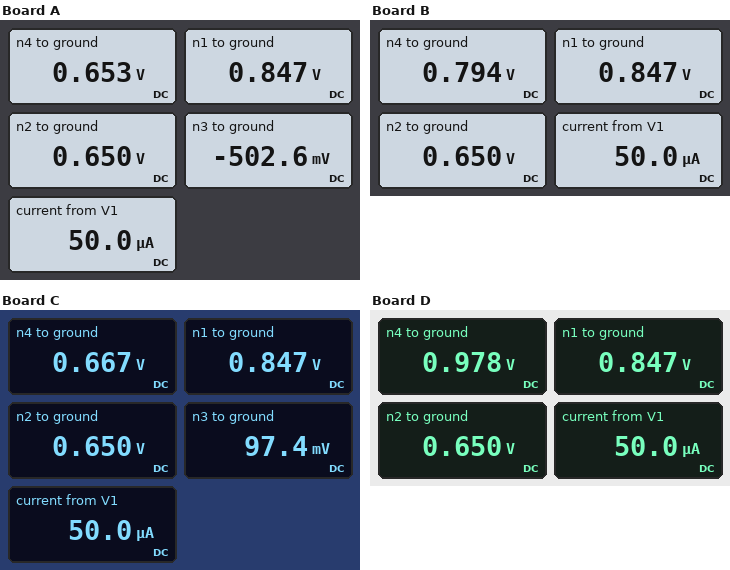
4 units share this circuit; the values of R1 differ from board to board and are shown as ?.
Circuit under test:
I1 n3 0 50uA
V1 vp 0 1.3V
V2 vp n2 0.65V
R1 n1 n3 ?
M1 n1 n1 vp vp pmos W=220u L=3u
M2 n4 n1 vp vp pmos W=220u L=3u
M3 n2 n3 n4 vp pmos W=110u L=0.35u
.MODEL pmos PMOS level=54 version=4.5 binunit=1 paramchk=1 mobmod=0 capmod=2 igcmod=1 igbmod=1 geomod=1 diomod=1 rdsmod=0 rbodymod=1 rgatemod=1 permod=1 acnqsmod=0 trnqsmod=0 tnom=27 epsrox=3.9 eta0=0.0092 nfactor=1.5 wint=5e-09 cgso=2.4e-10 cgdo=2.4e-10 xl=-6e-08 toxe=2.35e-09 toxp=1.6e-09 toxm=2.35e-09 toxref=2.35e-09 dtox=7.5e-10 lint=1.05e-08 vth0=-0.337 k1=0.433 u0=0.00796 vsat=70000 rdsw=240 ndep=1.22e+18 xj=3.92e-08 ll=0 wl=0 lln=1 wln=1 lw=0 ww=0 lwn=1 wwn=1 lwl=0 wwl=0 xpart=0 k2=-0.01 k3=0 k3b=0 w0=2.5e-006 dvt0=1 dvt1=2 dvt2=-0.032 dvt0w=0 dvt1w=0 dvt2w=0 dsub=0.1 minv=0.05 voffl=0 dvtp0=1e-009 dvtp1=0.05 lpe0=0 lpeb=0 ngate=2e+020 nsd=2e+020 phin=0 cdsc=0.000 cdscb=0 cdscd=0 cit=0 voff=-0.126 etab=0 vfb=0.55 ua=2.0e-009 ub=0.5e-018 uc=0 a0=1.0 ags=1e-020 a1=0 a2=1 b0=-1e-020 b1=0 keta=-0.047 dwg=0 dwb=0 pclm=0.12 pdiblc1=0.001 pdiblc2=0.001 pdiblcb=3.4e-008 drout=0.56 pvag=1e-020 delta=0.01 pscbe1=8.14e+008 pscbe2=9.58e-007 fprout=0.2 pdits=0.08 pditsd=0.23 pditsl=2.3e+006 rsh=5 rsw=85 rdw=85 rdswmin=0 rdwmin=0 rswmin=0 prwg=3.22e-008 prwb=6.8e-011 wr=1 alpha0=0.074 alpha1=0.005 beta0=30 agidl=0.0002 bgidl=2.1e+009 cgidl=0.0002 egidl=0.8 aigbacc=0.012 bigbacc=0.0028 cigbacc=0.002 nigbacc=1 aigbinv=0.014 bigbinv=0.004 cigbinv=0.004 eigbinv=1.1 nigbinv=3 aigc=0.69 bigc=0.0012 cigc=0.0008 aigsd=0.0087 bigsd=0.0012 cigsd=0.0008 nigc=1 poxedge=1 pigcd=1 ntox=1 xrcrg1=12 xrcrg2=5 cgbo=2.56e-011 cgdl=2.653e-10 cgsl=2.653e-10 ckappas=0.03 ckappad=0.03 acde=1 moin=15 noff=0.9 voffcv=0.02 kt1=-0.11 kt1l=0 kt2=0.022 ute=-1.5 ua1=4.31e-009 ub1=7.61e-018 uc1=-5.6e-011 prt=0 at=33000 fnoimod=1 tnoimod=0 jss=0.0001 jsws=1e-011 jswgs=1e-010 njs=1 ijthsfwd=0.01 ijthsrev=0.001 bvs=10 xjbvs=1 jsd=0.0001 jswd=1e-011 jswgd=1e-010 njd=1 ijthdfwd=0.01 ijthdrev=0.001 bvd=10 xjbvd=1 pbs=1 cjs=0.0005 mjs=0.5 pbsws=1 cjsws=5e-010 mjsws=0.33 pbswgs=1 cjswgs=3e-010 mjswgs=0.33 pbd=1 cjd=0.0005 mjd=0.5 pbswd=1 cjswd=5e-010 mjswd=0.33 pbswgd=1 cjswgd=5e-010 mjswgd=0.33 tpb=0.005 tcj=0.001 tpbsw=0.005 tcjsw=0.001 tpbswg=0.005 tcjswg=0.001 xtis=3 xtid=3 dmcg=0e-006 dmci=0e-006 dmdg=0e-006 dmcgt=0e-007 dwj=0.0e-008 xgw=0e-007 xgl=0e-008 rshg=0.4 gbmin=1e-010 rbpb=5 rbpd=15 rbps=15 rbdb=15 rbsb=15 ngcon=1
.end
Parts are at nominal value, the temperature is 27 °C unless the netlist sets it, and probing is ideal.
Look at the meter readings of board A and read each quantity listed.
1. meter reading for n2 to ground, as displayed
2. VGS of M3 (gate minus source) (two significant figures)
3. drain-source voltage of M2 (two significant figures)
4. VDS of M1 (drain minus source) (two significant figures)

0.650 V
-1.2 V
-650 mV
-450 mV
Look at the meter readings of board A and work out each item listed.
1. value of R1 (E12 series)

27 kΩ
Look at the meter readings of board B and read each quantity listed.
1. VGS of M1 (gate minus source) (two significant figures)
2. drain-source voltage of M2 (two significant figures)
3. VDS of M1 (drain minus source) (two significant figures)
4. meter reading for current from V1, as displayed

-450 mV
-510 mV
-450 mV
50.0 µA
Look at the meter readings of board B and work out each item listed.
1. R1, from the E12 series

10 kΩ
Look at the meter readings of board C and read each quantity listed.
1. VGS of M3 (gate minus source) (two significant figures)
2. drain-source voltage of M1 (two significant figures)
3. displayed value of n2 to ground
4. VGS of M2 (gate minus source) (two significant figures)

-570 mV
-450 mV
0.650 V
-450 mV
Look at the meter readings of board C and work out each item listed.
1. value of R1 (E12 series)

15 kΩ
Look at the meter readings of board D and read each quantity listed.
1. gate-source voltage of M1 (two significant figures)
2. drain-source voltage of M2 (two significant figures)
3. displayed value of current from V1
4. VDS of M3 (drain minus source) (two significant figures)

-450 mV
-320 mV
50.0 µA
-330 mV
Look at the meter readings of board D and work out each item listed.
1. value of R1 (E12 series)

5.6 kΩ
